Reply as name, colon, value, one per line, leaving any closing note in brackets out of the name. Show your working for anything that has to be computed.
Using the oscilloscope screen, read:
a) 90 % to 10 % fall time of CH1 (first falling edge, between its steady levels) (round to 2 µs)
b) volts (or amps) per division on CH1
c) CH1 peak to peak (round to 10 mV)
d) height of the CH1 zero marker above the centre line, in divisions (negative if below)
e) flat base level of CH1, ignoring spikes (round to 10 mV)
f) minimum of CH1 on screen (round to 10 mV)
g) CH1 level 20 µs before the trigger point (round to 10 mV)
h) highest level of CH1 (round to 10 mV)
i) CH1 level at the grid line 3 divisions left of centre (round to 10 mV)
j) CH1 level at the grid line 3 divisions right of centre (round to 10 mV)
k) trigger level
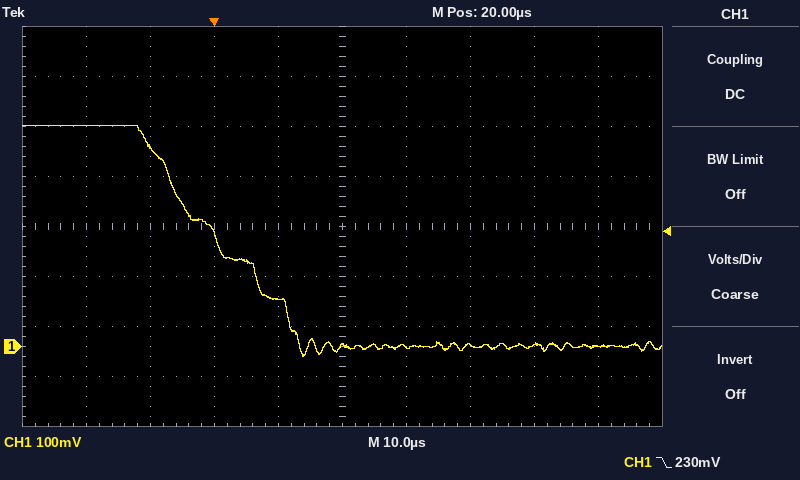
90 % to 10 % fall time of CH1 (first falling edge, between its steady levels): 22 µs
volts (or amps) per division on CH1: 100 mV
CH1 peak to peak: 440 mV − (-20 mV) = 460 mV
height of the CH1 zero marker above the centre line, in divisions: -2.4 div
flat base level of CH1, ignoring spikes: 0 mV
minimum of CH1 on screen: -20 mV
CH1 level 20 µs before the trigger point: 440 mV
highest level of CH1: 440 mV
CH1 level at the grid line 3 divisions left of centre: 400 mV
CH1 level at the grid line 3 divisions right of centre: 0 mV
trigger level: 230 mV
